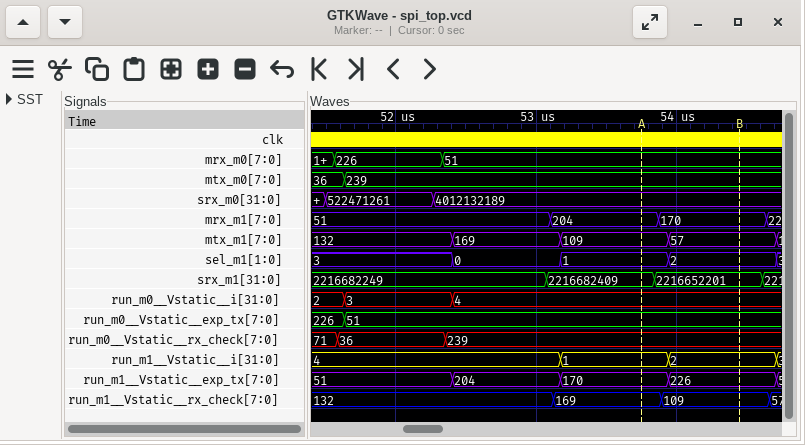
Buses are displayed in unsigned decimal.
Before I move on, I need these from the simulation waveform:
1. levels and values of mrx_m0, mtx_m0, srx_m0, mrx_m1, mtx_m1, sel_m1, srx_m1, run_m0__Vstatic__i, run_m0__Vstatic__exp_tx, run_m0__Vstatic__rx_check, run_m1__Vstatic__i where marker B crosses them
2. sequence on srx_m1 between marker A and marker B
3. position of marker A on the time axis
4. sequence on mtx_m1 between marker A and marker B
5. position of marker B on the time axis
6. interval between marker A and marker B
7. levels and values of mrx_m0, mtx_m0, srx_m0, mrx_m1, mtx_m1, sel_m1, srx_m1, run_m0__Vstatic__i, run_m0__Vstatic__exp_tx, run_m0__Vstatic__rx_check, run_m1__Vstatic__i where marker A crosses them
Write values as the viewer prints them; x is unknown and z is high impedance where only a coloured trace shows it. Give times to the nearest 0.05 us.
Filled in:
mrx_m0=51, mtx_m0=239, srx_m0=4012132189, mrx_m1=170, mtx_m1=57, sel_m1=2, srx_m1=2216652201, run_m0__Vstatic__i=4, run_m0__Vstatic__exp_tx=51, run_m0__Vstatic__rx_check=239, run_m1__Vstatic__i=2
2216682409, 2216652201
53.75 us
109, 57
54.45 us
0.7 us
mrx_m0=51, mtx_m0=239, srx_m0=4012132189, mrx_m1=204, mtx_m1=109, sel_m1=1, srx_m1=2216682409, run_m0__Vstatic__i=4, run_m0__Vstatic__exp_tx=51, run_m0__Vstatic__rx_check=239, run_m1__Vstatic__i=1
